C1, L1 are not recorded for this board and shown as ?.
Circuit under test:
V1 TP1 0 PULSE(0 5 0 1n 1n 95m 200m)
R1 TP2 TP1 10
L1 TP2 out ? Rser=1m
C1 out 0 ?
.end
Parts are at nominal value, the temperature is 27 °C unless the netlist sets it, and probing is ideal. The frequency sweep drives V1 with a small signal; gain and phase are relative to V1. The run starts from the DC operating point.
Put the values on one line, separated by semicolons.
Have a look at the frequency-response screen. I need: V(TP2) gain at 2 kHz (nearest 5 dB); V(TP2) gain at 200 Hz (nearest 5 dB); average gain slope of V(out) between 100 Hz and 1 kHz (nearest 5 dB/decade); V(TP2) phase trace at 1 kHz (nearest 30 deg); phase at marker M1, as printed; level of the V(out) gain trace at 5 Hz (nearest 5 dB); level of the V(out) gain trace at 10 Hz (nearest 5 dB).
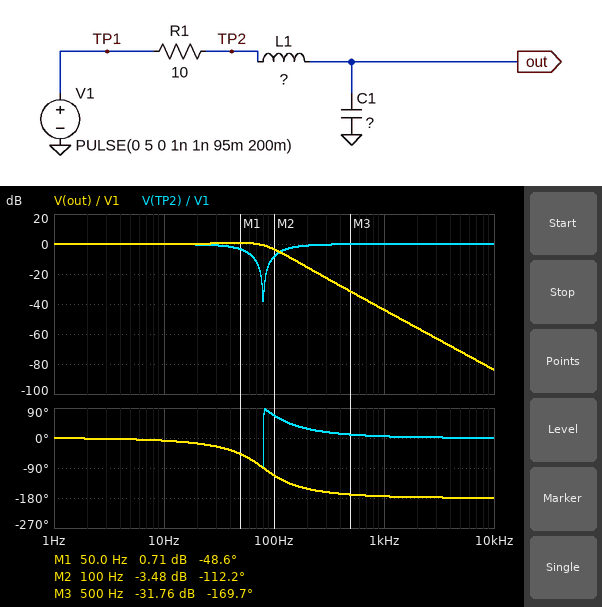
0 dB; 0 dB; -40 dB/decade; 0 deg; -48.6 deg; 0 dB; 0 dB
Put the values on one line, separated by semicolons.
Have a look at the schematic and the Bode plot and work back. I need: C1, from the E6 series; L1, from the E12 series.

220 µF; 18 mH
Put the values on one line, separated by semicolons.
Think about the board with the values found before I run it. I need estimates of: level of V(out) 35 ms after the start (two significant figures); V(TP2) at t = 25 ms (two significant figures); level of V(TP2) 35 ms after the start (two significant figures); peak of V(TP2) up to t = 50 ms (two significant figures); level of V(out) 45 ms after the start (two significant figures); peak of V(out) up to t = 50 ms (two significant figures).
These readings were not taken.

5.0 V; 5.0 V; 5.0 V; 5.4 V; 5.0 V; 5.6 V
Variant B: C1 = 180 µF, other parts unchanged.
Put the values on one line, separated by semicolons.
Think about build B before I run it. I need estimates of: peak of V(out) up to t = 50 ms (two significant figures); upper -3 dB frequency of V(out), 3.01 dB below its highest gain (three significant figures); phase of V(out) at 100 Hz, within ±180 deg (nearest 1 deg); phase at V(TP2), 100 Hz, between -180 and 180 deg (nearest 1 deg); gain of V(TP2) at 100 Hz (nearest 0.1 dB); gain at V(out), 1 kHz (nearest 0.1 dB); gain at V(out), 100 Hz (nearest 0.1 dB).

5.8 V; 103 Hz; -104 deg; 76 deg; -12.4 dB; -42.1 dB; -1.3 dB
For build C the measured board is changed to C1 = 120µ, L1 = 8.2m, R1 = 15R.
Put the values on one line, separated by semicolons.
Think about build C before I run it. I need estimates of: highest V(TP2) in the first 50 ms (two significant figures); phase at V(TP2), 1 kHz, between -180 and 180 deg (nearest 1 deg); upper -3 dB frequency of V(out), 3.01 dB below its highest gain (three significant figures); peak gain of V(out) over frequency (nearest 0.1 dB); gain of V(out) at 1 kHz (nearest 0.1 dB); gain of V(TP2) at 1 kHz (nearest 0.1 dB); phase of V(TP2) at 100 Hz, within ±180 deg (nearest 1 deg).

5.0 V; 17 deg; 118 Hz; 0 dB; -31.9 dB; -0.4 dB; -62 deg
